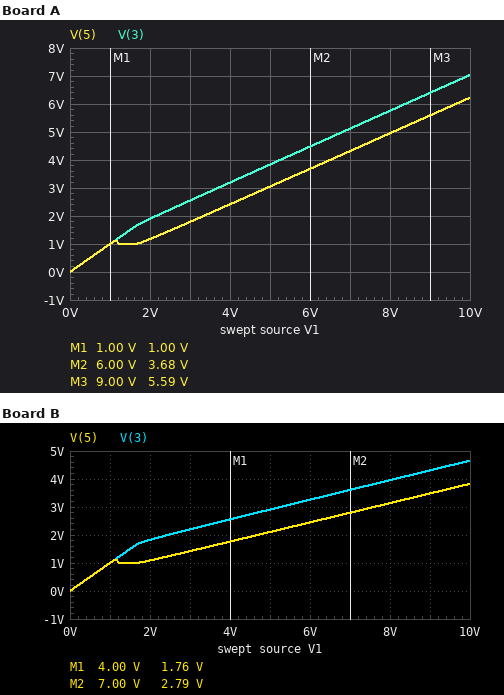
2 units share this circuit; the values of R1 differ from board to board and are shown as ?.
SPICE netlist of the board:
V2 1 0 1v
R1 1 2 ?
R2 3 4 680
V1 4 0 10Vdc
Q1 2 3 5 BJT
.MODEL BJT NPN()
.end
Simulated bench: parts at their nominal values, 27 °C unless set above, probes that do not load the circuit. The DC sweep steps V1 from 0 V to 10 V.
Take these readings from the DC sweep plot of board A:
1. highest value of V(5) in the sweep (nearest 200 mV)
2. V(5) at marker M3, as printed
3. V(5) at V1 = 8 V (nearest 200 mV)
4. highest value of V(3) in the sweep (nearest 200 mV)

6.2 V
5.59 V
5.0 V
7.0 V
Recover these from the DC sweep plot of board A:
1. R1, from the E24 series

1.2 kΩ
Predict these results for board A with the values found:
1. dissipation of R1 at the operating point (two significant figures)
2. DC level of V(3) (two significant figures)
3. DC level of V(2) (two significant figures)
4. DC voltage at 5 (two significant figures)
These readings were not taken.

23 mW
7.0 V
6.2 V
6.2 V
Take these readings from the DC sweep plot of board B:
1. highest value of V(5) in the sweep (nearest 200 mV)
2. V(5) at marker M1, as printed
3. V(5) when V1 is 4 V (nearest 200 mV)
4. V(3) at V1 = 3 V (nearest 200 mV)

3.8 V
1.76 V
1.8 V
2.2 V
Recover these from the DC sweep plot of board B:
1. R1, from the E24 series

360 Ω
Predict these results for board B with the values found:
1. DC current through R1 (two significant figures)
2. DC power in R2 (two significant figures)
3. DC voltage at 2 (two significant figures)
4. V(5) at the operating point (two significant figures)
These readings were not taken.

7.9 mA
42 mW
3.8 V
3.8 V
